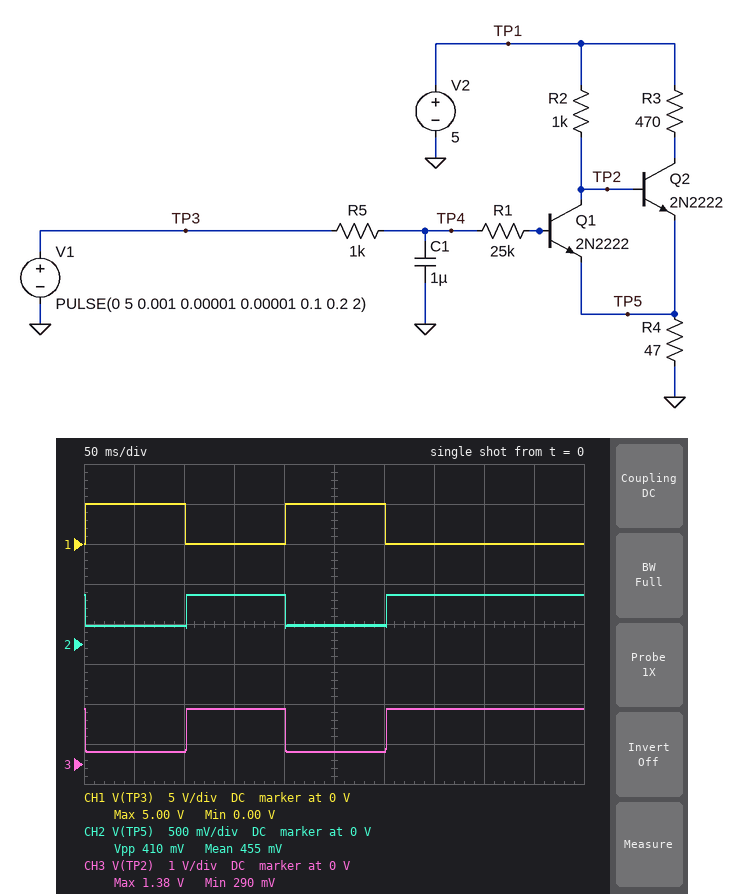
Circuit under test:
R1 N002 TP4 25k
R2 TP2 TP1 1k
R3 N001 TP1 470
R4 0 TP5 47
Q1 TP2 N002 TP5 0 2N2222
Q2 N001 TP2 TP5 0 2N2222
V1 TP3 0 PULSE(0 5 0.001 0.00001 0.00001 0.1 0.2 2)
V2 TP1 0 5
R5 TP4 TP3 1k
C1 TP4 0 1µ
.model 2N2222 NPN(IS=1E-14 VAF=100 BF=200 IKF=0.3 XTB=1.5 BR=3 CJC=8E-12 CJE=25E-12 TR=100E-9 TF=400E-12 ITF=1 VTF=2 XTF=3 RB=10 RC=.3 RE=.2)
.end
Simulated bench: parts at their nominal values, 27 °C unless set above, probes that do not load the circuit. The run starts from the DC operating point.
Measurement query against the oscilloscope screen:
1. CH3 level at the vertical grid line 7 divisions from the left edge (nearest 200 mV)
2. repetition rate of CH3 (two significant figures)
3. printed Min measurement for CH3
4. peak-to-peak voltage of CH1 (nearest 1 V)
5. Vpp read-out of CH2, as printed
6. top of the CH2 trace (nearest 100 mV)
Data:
1.4 V
5.0 Hz
290 mV
5 V
410 mV
600 mV
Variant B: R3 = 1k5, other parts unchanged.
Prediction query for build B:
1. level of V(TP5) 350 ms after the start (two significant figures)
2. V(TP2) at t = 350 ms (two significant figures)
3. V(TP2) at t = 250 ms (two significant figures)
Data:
330 mV
1.1 V
300 mV
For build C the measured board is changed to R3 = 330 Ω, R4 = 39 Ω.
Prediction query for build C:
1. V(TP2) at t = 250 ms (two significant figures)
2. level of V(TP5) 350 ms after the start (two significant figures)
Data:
260 mV
650 mV
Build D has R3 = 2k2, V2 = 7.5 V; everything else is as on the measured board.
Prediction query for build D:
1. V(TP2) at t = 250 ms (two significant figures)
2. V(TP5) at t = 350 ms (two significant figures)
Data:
420 mV
440 mV
